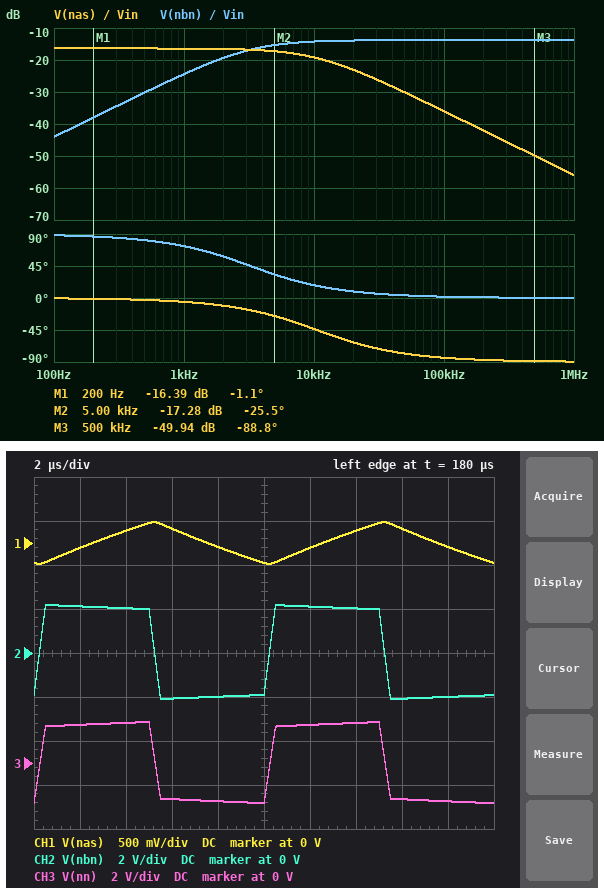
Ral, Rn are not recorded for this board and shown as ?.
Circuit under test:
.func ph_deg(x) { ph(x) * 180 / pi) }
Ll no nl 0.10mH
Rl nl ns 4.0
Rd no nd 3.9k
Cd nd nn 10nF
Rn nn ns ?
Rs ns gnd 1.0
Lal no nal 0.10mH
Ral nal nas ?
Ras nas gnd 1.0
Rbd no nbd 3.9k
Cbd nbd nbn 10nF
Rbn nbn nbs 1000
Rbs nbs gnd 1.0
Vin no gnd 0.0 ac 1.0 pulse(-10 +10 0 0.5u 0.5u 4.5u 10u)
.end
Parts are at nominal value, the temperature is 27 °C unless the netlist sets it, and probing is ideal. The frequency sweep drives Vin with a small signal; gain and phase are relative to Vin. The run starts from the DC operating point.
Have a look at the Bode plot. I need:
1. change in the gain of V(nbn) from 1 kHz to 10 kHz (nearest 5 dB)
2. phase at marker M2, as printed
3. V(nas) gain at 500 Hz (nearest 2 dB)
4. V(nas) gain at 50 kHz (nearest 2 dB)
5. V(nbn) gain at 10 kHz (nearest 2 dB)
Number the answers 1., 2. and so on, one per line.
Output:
1. 10 dB
2. -25.5 deg
3. -16 dB
4. -30 dB
5. -14 dB
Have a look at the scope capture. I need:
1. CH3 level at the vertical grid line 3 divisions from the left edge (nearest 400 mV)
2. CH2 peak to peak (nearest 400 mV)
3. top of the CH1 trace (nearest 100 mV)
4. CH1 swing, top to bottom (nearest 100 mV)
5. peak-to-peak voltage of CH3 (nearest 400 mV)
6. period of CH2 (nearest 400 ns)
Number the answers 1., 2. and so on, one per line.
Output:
1. -1.6 V
2. 4.4 V
3. 200 mV
4. 500 mV
5. 3.6 V
6. 10.0 µs
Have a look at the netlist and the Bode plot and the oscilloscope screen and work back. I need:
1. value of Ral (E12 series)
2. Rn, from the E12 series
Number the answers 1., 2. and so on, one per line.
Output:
1. 5.6 Ω
2. 820 Ω
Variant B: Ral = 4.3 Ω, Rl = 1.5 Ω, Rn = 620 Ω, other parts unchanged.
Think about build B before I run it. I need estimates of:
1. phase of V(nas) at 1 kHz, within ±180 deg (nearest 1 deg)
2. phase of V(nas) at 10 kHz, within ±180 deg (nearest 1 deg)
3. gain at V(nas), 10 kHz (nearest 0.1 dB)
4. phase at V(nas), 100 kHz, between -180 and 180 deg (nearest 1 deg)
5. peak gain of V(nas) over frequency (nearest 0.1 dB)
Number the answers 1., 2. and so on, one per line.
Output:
1. -7 deg
2. -50 deg
3. -18.3 dB
4. -85 deg
5. -14.5 dB
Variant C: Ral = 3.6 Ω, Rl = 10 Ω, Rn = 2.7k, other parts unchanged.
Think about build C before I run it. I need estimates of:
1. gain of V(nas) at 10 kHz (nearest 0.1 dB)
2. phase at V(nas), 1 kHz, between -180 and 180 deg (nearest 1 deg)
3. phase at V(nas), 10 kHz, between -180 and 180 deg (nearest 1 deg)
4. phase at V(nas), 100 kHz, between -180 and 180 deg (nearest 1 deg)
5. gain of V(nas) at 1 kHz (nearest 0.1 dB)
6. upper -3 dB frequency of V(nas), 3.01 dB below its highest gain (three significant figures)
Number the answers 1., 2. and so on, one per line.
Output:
1. -17.8 dB
2. -8 deg
3. -54 deg
4. -86 deg
5. -13.3 dB
6. 7.32 kHz
